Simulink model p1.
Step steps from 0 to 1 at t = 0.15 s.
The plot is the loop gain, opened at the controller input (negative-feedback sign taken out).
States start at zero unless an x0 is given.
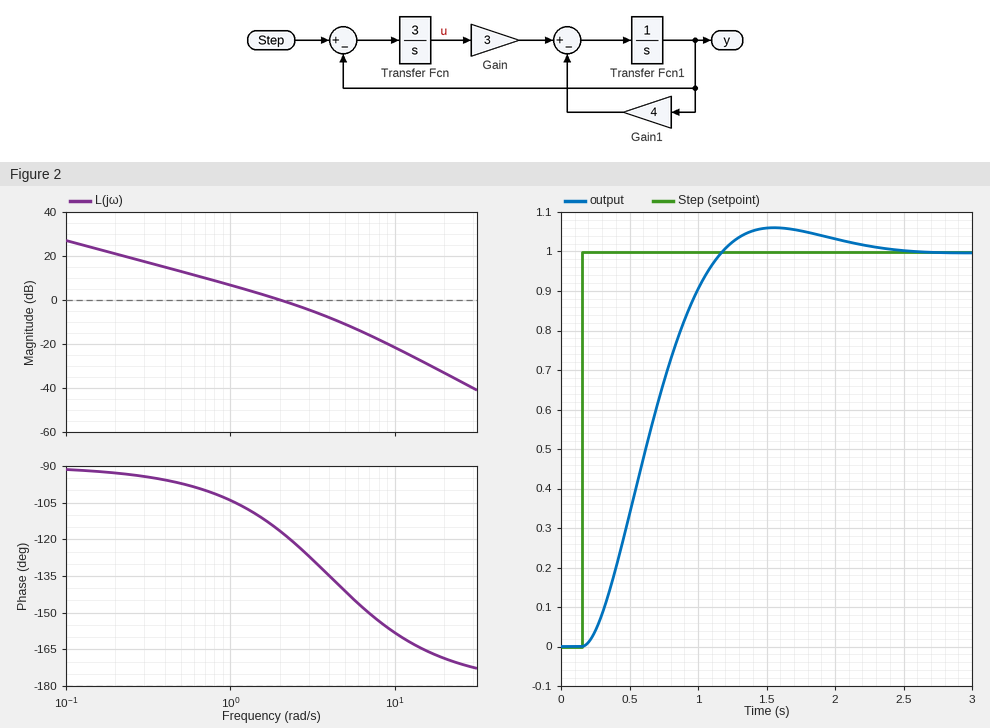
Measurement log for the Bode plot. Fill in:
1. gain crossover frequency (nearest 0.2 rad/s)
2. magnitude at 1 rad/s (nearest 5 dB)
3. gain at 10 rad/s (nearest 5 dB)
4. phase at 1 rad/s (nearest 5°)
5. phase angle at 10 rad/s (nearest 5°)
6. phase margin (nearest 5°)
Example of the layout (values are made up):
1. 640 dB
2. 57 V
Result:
1. 2.0 rad/s
2. 5 dB
3. -20 dB
4. -105°
5. -160°
6. 65°
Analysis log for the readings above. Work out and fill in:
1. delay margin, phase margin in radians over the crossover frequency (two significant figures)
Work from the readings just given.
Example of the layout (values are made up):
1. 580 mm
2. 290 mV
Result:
1. 0.57 s
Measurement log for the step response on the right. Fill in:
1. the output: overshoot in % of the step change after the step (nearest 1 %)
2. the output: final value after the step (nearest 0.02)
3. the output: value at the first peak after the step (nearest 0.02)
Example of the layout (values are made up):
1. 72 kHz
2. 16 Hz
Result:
1. 6 %
2. 1.00
3. 1.06
